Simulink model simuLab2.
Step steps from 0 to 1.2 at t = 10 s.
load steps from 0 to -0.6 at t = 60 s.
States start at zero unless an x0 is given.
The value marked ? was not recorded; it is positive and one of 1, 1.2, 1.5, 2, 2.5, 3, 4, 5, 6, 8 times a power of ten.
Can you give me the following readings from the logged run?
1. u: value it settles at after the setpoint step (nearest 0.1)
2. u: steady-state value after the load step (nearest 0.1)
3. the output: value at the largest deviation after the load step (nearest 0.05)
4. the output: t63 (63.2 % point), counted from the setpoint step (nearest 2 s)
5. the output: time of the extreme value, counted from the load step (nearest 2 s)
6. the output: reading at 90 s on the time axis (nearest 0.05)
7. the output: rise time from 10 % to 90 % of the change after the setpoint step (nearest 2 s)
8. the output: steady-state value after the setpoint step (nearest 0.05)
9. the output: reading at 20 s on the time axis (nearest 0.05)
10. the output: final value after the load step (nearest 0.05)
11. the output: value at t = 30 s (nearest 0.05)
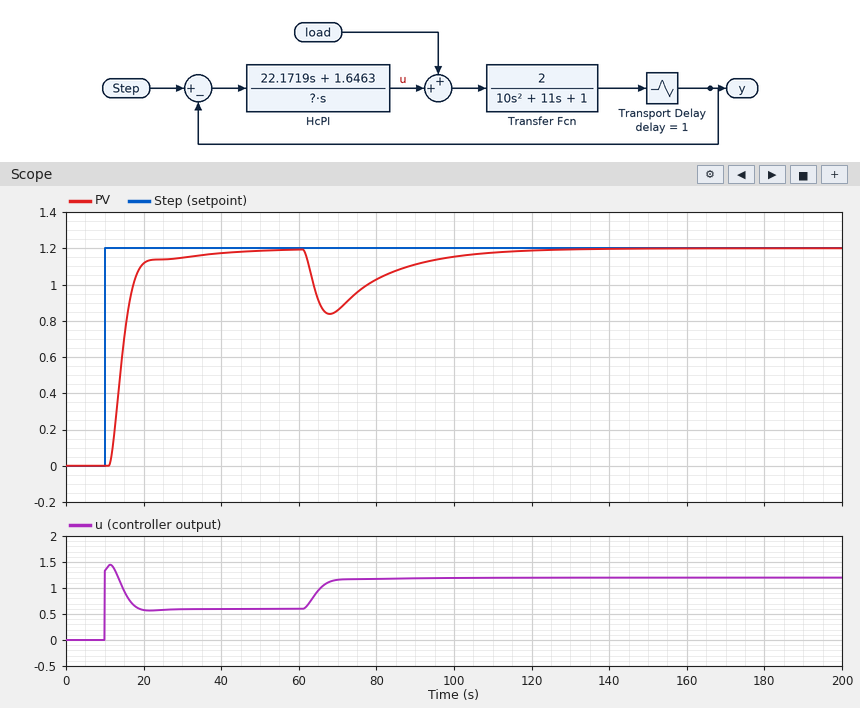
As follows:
0.6
1.2
0.85
6 s
8 s
1.10
6 s
1.20
1.10
1.20
1.15
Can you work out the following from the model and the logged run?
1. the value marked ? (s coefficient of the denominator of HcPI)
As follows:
20
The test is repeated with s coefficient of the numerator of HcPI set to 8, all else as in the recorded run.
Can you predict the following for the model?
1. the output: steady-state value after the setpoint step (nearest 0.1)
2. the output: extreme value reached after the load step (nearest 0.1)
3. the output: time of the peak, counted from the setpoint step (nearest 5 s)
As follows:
1.2
0.7
25 s
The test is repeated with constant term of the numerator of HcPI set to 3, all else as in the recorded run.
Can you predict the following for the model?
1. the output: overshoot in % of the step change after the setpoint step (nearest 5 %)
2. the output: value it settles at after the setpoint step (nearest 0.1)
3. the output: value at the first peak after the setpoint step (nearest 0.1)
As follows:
10 %
1.2
1.3
